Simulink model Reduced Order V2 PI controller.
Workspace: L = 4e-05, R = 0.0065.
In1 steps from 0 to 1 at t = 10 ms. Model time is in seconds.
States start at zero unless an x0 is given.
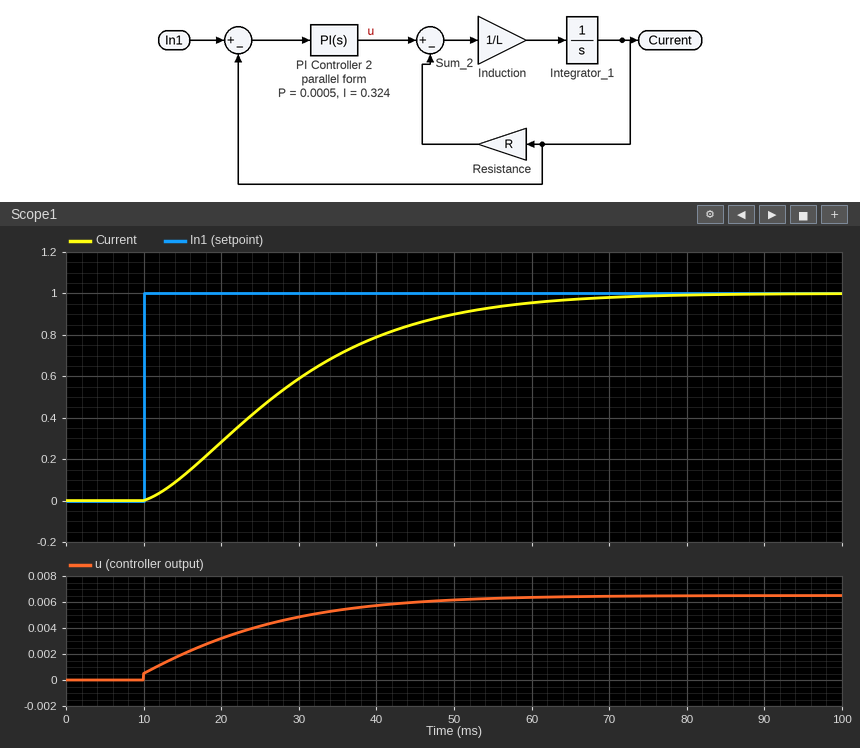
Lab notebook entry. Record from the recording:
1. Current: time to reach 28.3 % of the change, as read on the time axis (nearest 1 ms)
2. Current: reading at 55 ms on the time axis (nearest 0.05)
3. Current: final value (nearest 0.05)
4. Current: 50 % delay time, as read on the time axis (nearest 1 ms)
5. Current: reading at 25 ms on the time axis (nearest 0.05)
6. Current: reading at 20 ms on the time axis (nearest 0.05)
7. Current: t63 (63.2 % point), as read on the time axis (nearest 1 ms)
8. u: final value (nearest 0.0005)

20 ms
0.95
1.00
27 ms
0.45
0.30
32 ms
0.0065
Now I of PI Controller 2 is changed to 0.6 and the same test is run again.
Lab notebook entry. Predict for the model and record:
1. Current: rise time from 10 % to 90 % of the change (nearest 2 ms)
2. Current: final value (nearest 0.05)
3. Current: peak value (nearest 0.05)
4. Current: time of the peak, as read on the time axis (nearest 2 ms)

18 ms
1.00
1.05
46 ms
